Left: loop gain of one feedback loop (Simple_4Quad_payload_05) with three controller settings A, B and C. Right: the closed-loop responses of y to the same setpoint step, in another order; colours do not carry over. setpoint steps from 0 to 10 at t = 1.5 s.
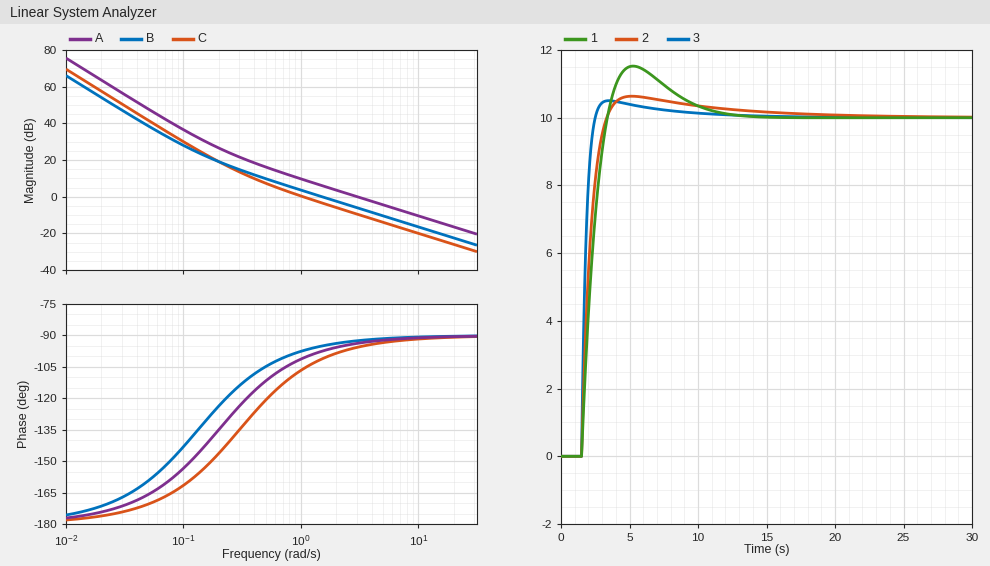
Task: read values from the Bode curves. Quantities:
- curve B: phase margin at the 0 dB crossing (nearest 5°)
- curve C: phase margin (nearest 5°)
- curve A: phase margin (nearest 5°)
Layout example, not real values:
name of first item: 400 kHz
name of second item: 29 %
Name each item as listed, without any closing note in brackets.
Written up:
curve B: phase margin at the 0 dB crossing: 85°
curve C: phase margin: 75°
curve A: phase margin: 85°
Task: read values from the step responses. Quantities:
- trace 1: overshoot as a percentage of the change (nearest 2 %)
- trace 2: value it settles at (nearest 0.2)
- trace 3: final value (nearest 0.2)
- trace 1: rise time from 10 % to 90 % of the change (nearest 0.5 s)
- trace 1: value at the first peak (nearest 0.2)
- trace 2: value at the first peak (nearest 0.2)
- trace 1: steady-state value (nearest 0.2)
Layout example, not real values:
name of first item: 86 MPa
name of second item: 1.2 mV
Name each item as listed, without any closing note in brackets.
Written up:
trace 1: overshoot as a percentage of the change: 16 %
trace 2: value it settles at: 10.0
trace 3: final value: 10.0
trace 1: rise time from 10 % to 90 % of the change: 1.5 s
trace 1: value at the first peak: 11.6
trace 2: value at the first peak: 10.6
trace 1: steady-state value: 10.0
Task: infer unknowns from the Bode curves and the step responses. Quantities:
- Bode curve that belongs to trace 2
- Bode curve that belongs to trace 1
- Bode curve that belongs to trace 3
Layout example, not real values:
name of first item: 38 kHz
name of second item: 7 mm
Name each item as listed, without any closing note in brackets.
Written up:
Bode curve that belongs to trace 2: B
Bode curve that belongs to trace 1: C
Bode curve that belongs to trace 3: A
